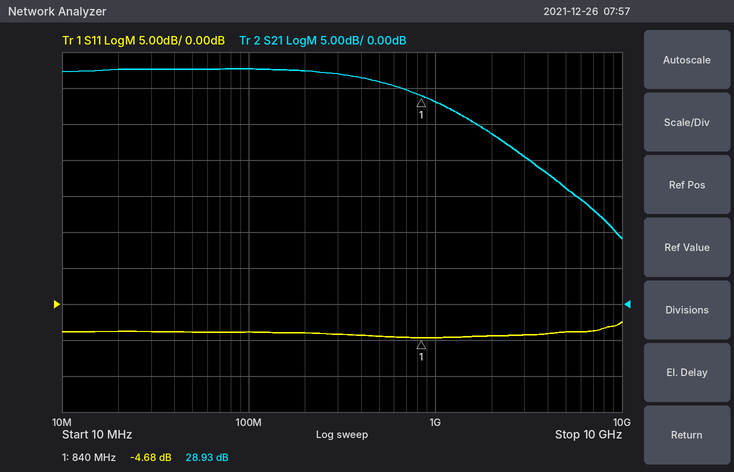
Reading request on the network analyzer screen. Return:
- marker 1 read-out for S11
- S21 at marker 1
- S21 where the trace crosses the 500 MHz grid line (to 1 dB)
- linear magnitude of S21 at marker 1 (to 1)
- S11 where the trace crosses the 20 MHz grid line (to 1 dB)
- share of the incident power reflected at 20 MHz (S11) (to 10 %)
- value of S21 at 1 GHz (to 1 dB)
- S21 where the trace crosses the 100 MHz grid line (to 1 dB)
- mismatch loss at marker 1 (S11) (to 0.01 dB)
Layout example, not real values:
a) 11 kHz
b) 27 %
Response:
a) -4.68 dB
b) 28.93 dB
c) 31 dB
d) 28
e) -4 dB
f) 40 %
g) 28 dB
h) 33 dB
i) 1.81 dB
